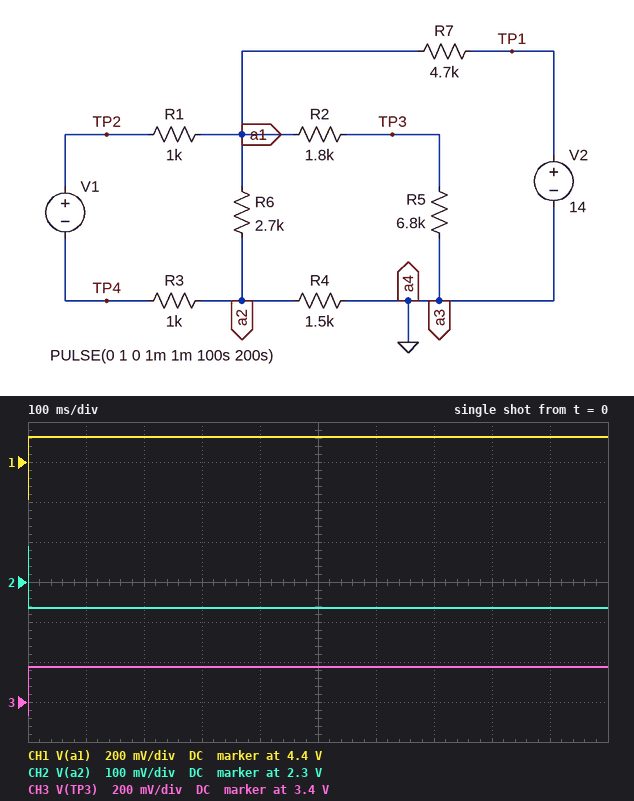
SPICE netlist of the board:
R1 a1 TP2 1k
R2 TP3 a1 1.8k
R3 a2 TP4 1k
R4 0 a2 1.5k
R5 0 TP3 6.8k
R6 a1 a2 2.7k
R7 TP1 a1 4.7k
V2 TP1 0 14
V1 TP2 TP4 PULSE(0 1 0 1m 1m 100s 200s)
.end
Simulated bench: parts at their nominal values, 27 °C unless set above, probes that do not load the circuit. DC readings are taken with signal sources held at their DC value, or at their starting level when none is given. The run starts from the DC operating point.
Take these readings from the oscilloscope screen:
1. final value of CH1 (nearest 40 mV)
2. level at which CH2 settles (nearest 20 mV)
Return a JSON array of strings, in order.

["4.52 V", "2.24 V"]
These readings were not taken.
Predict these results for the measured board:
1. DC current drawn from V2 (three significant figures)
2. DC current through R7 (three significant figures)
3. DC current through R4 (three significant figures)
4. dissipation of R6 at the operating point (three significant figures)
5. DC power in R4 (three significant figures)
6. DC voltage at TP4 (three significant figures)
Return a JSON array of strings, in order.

["2.08 mA", "2.08 mA", "1.59 mA", "1.24 mW", "3.80 mW", "3.30 V"]
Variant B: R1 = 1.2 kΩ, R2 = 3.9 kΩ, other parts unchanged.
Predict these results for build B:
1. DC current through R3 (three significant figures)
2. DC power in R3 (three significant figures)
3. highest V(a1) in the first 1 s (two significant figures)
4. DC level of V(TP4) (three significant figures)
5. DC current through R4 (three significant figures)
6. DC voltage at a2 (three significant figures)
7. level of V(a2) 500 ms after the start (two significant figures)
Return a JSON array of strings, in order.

["897 µA", "804 µW", "4.7 V", "3.34 V", "1.63 mA", "2.44 V", "2.3 V"]
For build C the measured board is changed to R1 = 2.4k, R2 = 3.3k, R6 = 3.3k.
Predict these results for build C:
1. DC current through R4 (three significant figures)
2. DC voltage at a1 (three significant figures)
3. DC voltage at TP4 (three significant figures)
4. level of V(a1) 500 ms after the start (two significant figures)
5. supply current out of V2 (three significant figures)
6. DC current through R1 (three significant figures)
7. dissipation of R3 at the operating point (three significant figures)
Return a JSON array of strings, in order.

["1.50 mA", "4.75 V", "2.98 V", "5.0 V", "1.97 mA", "737 µA", "544 µW"]
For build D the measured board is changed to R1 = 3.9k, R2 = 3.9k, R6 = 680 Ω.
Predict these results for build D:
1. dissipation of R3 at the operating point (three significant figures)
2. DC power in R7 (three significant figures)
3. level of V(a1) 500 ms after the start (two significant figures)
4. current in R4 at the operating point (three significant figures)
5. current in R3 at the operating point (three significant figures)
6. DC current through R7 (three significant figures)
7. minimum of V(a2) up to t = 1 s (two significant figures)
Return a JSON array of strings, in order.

["48.9 µW", "22.1 mW", "3.9 V", "1.81 mA", "221 µA", "2.17 mA", "2.7 V"]
